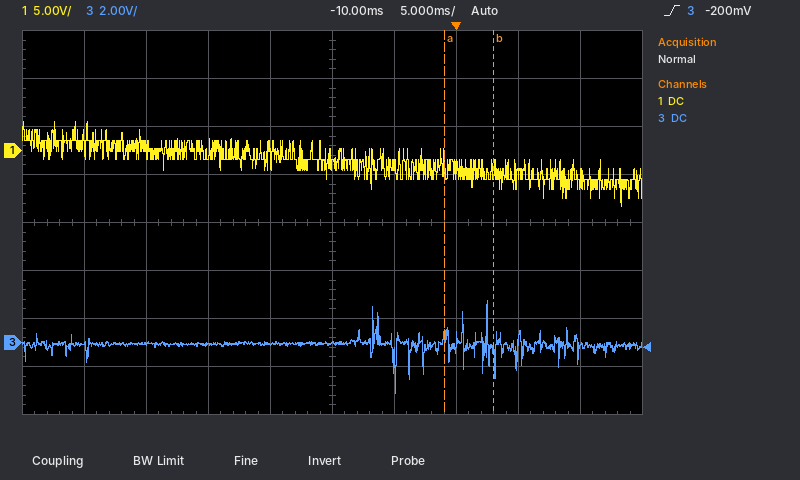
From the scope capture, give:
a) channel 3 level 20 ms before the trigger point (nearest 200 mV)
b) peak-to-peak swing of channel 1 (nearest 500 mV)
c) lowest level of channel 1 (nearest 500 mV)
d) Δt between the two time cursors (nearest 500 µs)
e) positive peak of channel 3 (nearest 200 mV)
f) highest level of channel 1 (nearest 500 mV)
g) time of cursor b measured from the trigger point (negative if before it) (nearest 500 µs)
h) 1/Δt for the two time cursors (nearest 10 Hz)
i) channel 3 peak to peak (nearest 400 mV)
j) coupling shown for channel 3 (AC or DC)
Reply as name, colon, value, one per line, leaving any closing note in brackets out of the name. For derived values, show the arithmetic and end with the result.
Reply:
channel 3 level 20 ms before the trigger point: 0.0 V
peak-to-peak swing of channel 1: 3.0 V − (-6.0 V) = 9.0 V
lowest level of channel 1: -6.0 V
Δt between the two time cursors: 4.0 ms
positive peak of channel 3: 1.8 V
highest level of channel 1: 3.0 V
time of cursor b measured from the trigger point (negative if before it): +3.0 ms
1/Δt for the two time cursors: 1 / 4.0 ms ≈ 250 Hz
channel 3 peak to peak: 4.0 V
coupling shown for channel 3: DC
